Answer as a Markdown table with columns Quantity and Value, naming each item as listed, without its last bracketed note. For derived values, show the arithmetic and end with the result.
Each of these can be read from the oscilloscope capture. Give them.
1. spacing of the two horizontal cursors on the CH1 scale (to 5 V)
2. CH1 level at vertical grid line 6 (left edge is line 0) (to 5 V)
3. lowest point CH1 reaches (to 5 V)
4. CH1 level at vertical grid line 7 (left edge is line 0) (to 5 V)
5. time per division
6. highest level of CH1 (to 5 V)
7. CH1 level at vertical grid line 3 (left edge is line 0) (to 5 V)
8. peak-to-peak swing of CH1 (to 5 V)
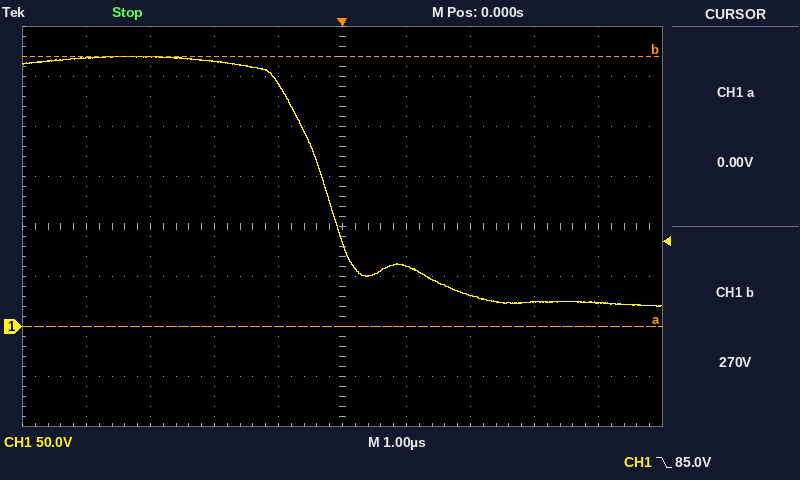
| Quantity | Value |
|---|---|
| spacing of the two horizontal cursors on the CH1 scale | 270 V |
| CH1 level at vertical grid line 6 (left edge is line 0) | 60 V |
| lowest point CH1 reaches | 20 V |
| CH1 level at vertical grid line 7 (left edge is line 0) | 30 V |
| time per division | 1 µs |
| highest level of CH1 | 270 V |
| CH1 level at vertical grid line 3 (left edge is line 0) | 265 V |
| peak-to-peak swing of CH1 | 270 V − (20 V) = 250 V |
